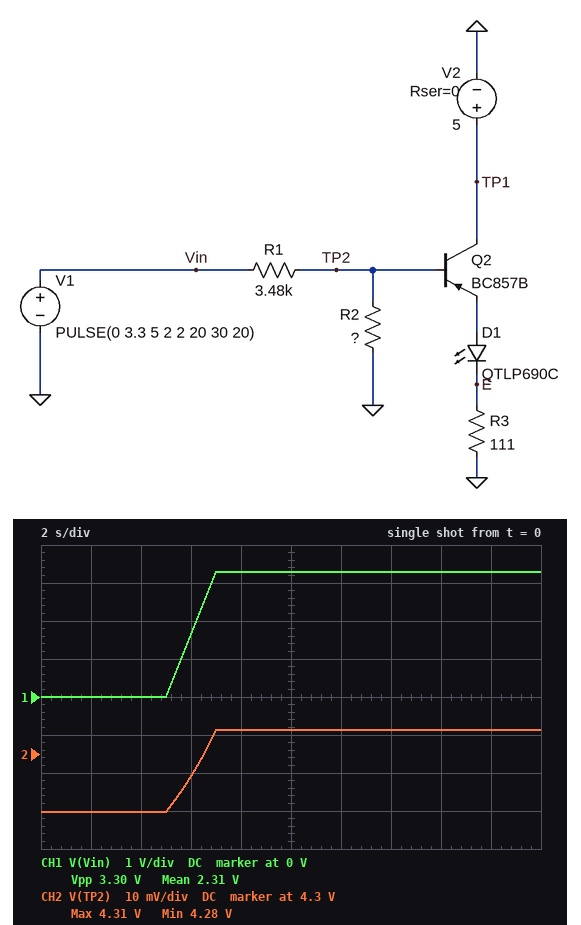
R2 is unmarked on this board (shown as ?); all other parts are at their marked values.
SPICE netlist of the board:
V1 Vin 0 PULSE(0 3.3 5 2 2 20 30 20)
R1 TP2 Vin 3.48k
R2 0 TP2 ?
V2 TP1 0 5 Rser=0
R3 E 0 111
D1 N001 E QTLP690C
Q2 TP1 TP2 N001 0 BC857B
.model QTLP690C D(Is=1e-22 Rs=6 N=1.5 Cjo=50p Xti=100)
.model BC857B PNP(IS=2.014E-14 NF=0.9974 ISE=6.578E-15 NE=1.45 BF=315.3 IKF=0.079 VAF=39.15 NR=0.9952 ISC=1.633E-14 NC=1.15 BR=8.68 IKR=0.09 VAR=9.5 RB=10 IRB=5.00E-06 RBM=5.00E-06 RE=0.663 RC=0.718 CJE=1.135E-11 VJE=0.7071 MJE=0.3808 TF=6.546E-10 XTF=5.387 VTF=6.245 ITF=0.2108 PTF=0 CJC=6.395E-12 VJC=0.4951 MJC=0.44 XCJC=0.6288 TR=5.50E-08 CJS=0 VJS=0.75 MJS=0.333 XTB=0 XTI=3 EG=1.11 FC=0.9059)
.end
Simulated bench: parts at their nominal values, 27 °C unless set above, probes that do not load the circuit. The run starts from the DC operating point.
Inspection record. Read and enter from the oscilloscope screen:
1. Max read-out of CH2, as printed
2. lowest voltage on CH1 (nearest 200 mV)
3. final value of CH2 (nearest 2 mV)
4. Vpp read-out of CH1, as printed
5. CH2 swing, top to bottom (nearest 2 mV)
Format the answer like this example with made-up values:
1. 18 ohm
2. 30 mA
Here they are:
1. 4.31 V
2. 0 V
3. 4.306 V
4. 3.30 V
5. 22 mV
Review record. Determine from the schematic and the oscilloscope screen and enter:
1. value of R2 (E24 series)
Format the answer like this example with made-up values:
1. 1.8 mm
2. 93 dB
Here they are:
1. 5.6 kΩ
